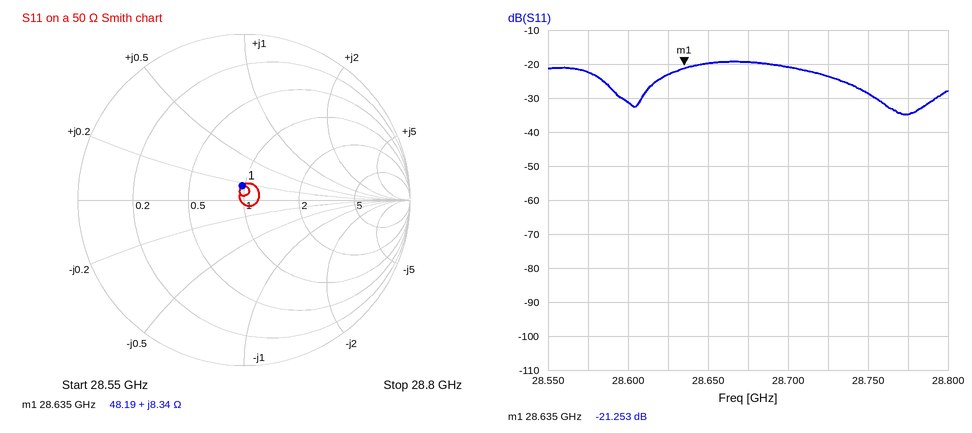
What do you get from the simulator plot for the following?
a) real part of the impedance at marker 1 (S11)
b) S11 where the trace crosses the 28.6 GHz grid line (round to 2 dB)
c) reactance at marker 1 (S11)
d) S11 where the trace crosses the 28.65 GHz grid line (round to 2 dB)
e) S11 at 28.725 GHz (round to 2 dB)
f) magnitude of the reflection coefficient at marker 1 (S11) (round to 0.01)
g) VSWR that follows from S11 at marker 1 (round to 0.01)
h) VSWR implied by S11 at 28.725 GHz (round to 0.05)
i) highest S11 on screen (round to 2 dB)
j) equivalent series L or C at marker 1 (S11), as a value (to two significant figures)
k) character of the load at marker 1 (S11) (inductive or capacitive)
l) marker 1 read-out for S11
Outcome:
48.19 Ω
-32 dB
+8.34 Ω
-20 dB
-24 dB
0.09
1.19
1.15
-20 dB
46 pH
inductive
-21.253 dB
